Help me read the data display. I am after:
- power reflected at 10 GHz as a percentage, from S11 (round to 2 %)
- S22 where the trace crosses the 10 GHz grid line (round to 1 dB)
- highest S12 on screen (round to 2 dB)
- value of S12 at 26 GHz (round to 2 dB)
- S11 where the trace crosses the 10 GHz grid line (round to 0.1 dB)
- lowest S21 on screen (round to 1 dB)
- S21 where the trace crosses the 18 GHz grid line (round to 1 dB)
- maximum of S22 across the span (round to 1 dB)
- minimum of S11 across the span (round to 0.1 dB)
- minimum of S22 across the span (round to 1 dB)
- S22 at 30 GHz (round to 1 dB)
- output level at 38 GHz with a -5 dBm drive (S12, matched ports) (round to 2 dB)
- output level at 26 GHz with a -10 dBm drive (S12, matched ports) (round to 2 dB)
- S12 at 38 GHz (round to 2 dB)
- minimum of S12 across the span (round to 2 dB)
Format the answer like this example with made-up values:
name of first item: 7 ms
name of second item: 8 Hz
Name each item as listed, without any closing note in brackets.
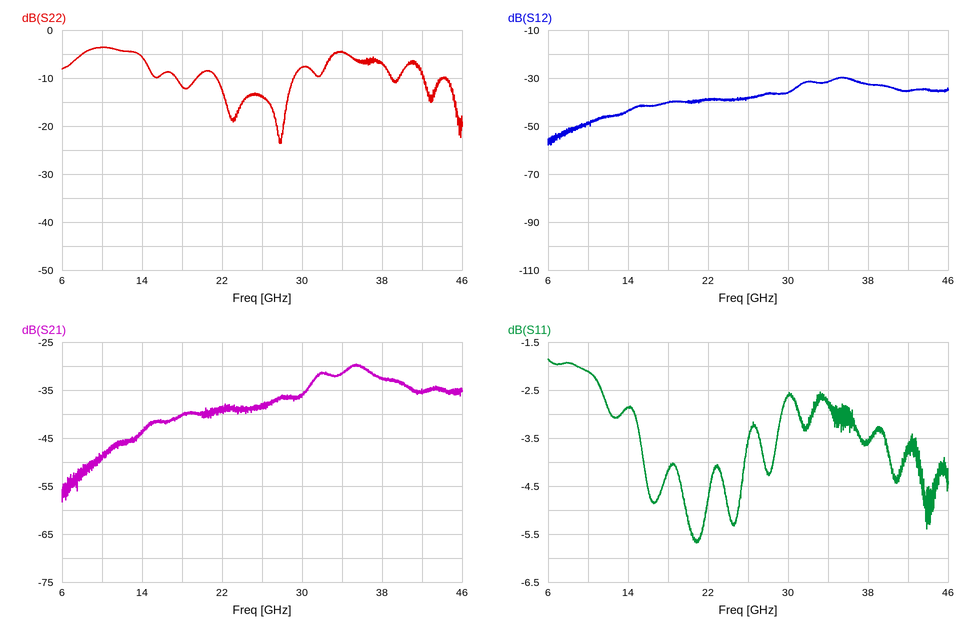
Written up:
power reflected at 10 GHz as a percentage, from S11: 62 %
S22 where the trace crosses the 10 GHz grid line: -4 dB
highest S12 on screen: -30 dB
value of S12 at 26 GHz: -38 dB
S11 where the trace crosses the 10 GHz grid line: -2.1 dB
lowest S21 on screen: -58 dB
S21 where the trace crosses the 18 GHz grid line: -40 dB
maximum of S22 across the span: -4 dB
minimum of S11 across the span: -5.7 dB
minimum of S22 across the span: -24 dB
S22 at 30 GHz: -8 dB
output level at 38 GHz with a -5 dBm drive (S12, matched ports): -38 dBm
output level at 26 GHz with a -10 dBm drive (S12, matched ports): -48 dBm
S12 at 38 GHz: -32 dB
minimum of S12 across the span: -58 dB
